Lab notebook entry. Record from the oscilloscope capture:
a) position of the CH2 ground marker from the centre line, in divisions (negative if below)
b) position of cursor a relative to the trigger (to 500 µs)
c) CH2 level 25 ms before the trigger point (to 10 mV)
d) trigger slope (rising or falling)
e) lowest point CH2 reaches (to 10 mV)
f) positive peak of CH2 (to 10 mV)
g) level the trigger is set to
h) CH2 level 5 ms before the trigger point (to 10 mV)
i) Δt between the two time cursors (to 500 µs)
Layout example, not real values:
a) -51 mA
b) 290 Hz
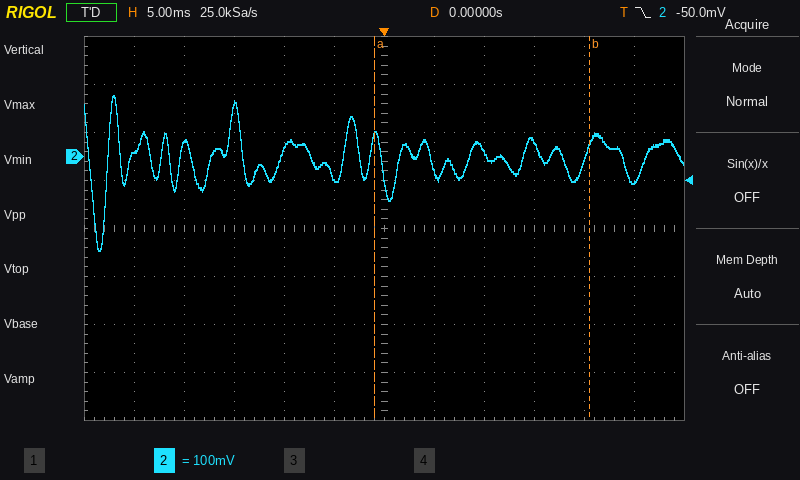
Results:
a) +1.5 div
b) -1.0 ms
c) 10 mV
d) falling
e) -200 mV
f) 130 mV
g) -50.0 mV
h) -40 mV
i) 21.5 ms
